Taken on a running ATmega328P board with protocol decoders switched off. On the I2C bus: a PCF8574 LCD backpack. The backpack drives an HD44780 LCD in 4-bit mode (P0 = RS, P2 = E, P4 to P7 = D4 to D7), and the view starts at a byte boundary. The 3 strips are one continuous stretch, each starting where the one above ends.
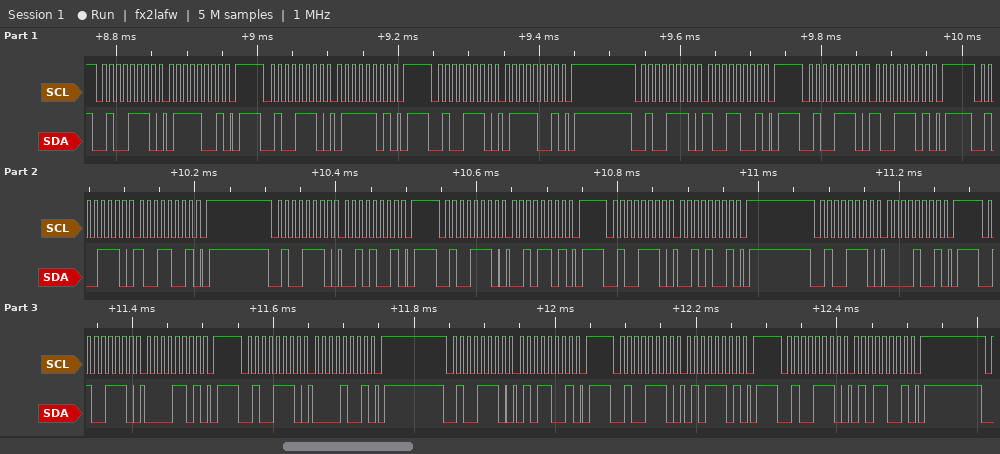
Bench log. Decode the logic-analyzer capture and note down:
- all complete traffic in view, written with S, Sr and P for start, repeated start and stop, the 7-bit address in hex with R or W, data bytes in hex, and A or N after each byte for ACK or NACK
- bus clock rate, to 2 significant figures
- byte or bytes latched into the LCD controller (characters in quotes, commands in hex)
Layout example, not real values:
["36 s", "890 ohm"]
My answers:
["S 27W A 79 A P S 27W A 7D A P S 27W A 79 A P S 27W A 99 A P S 27W A 9D A P S 27W A 99 A P S 27W A 29 A P S 27W A 2D A P S 27W A 29 A P S 27W A 09 A P S 27W A 0D A P S 27W A 09 A P S 27W A 59 A P S 27W A 5D A P S 27W A 59 A P", "100 kHz", "'y' ' '"]
